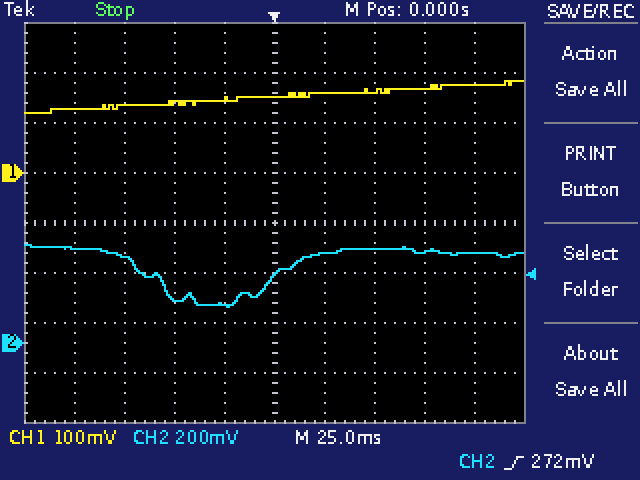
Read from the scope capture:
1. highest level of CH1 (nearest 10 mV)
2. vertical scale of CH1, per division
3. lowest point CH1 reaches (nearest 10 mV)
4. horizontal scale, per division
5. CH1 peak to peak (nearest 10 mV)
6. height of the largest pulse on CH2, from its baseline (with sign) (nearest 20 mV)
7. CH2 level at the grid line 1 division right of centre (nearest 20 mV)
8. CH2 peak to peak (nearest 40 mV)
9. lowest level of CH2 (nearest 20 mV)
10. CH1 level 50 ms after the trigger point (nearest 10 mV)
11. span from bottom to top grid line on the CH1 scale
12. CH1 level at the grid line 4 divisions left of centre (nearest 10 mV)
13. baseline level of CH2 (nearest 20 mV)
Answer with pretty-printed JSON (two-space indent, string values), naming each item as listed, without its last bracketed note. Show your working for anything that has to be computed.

{
  "highest level of CH1": "180 mV",
  "vertical scale of CH1, per division": "100 mV",
  "lowest point CH1 reaches": "120 mV",
  "horizontal scale, per division": "25 ms",
  "CH1 peak to peak": "180 mV − (120 mV) = 60 mV",
  "height of the largest pulse on CH2, from its baseline (with sign)": "140 mV − (360 mV) = -220 mV",
  "CH2 level at the grid line 1 division right of centre": "360 mV",
  "CH2 peak to peak": "240 mV",
  "lowest level of CH2": "140 mV",
  "CH1 level 50 ms after the trigger point": "160 mV",
  "span from bottom to top grid line on the CH1 scale": "800 mV",
  "CH1 level at the grid line 4 divisions left of centre": "130 mV",
  "baseline level of CH2": "360 mV"
}
